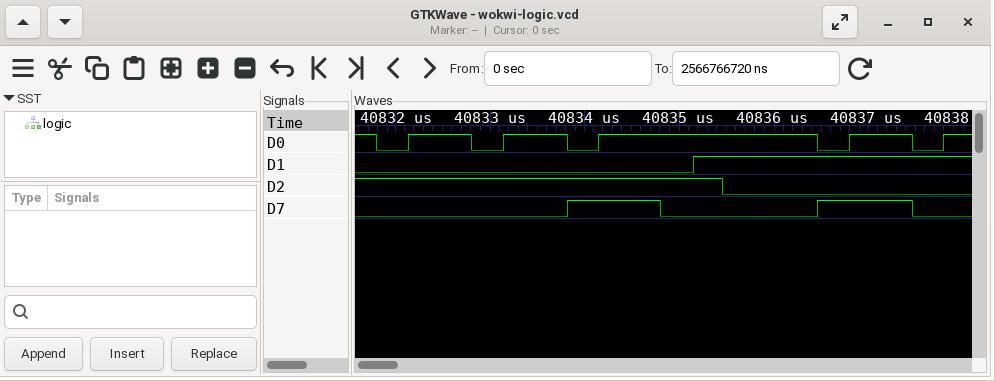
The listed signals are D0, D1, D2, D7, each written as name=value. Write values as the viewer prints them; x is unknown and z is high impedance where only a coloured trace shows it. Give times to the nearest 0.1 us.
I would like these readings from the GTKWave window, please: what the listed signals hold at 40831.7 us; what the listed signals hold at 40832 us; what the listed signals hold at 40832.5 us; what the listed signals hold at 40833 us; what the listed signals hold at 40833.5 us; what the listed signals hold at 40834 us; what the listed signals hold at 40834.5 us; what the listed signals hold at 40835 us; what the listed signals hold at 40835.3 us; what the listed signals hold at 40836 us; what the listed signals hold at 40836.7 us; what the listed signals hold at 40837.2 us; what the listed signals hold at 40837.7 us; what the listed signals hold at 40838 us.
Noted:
D0=1, D1=0, D2=1, D7=0
D0=0, D1=0, D2=1, D7=0
D0=1, D1=0, D2=1, D7=0
D0=0, D1=0, D2=1, D7=0
D0=1, D1=0, D2=1, D7=0
D0=0, D1=0, D2=1, D7=1
D0=1, D1=0, D2=1, D7=1
D0=1, D1=0, D2=1, D7=0
D0=1, D1=1, D2=1, D7=0
D0=1, D1=1, D2=0, D7=0
D0=0, D1=1, D2=0, D7=1
D0=1, D1=1, D2=0, D7=1
D0=0, D1=1, D2=0, D7=0
D0=1, D1=1, D2=0, D7=0
